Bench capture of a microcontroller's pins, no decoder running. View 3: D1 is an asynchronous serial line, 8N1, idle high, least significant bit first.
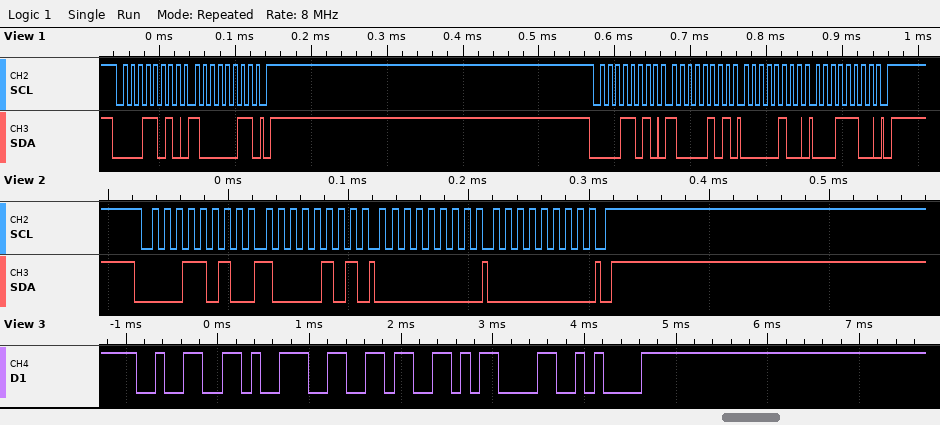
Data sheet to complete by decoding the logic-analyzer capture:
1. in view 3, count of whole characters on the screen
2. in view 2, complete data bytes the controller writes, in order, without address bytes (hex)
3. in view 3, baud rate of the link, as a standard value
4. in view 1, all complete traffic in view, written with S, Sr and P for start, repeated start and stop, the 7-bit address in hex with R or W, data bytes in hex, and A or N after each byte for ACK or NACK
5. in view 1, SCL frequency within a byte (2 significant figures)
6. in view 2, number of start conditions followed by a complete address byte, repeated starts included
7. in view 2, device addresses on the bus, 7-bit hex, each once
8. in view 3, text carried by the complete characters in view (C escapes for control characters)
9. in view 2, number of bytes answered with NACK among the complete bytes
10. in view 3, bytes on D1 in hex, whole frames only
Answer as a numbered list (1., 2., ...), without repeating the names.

1. 5
2. 85 00 00
3. 9600 baud
4. S 0DW A 83 A P S 0DW A 85 A 04 A 1C A P
5. 100 kHz
6. 1
7. 0x0D
8. "296\r\n"
9. 0
10. 32 39 36 0D 0A
